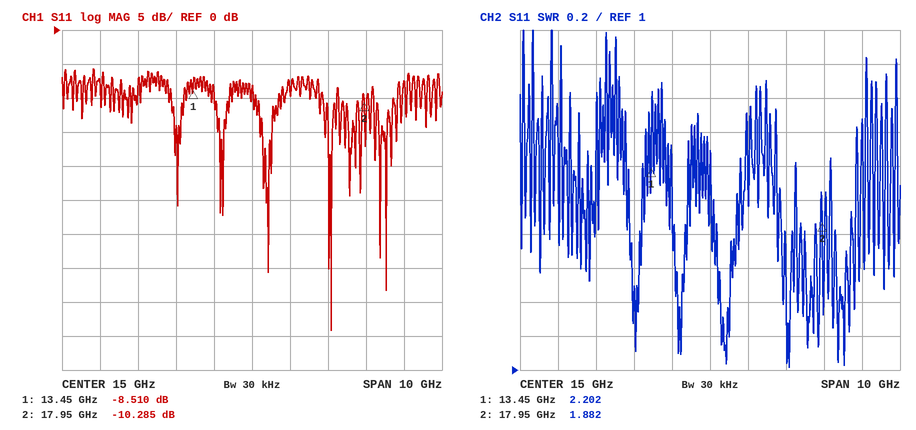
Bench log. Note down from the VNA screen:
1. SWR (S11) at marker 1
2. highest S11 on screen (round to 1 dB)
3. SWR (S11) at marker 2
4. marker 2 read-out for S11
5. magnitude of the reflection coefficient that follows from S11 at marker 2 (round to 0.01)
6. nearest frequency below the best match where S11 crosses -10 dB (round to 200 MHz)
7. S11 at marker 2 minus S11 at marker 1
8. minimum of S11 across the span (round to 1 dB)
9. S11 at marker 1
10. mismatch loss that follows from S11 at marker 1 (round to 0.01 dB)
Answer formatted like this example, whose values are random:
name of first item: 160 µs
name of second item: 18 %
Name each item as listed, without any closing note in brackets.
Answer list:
SWR (S11) at marker 1: 2.202
highest S11 on screen: -6 dB
SWR (S11) at marker 2: 1.882
marker 2 read-out for S11: -10.285 dB
magnitude of the reflection coefficient that follows from S11 at marker 2: 0.31
nearest frequency below the best match where S11 crosses -10 dB: 16.8 GHz
S11 at marker 2 minus S11 at marker 1: -1.775 dB
minimum of S11 across the span: -44 dB
S11 at marker 1: -8.510 dB
mismatch loss that follows from S11 at marker 1: 0.66 dB
